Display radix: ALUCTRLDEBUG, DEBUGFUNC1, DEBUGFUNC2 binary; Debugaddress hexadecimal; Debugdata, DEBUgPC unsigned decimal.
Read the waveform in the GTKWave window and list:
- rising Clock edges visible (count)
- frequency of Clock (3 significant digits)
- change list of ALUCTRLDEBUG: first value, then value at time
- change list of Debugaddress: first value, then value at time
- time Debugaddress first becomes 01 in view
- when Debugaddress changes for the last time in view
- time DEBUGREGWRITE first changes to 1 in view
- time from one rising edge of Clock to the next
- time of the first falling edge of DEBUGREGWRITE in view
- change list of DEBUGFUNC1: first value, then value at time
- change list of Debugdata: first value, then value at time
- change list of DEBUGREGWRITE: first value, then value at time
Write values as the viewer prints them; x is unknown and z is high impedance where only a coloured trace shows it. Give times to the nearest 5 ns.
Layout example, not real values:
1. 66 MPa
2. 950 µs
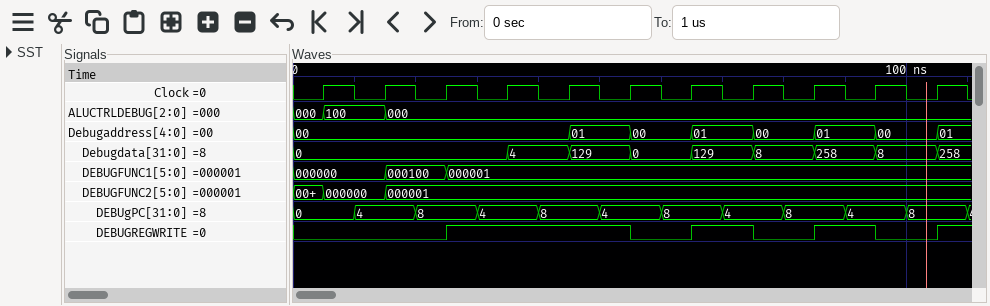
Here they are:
1. 11
2. 100 MHz
3. 000, 100 at 5 ns, 000 at 15 ns
4. 00, 01 at 45 ns, 00 at 55 ns, 01 at 65 ns, 00 at 75 ns, 01 at 85 ns, 00 at 95 ns, 01 at 105 ns
5. 45 ns
6. 105 ns
7. 25 ns
8. 10 ns
9. 55 ns
10. 000000, 000100 at 15 ns, 000001 at 25 ns
11. 0, 4 at 35 ns, 129 at 45 ns, 0 at 55 ns, 129 at 65 ns, 8 at 75 ns, 258 at 85 ns, 8 at 95 ns, 258 at 105 ns
12. 0, 1 at 25 ns, 0 at 55 ns, 1 at 65 ns, 0 at 75 ns, 1 at 85 ns, 0 at 95 ns, 1 at 105 ns
